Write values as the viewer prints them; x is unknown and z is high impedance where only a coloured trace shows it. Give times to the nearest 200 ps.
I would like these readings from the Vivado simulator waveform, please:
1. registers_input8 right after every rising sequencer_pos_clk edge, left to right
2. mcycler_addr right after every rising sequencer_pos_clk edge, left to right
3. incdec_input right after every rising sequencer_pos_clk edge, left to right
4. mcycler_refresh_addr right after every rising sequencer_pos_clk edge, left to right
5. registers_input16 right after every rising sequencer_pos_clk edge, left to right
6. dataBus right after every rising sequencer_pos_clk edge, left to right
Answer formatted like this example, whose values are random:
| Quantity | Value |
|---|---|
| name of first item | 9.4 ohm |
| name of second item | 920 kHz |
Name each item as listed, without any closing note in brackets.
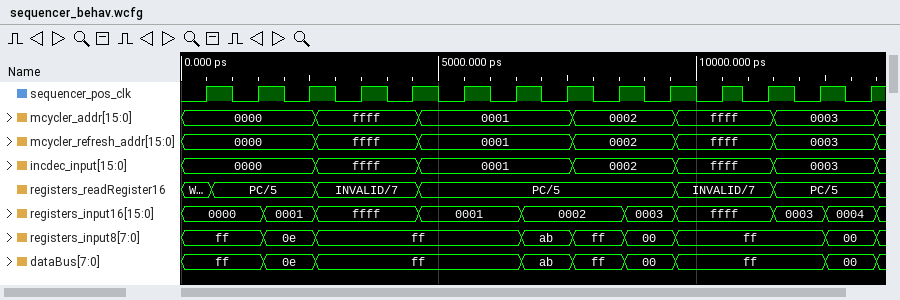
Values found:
| Quantity | Value |
|---|---|
| registers_input8 right after every rising sequencer_pos_clk edge, left to right | ff, ff, 0e, ff, ff, ff, ff, ab, ff, 00, ff, ff, ff, 00 |
| mcycler_addr right after every rising sequencer_pos_clk edge, left to right | 0000, 0000, 0000, ffff, ffff, 0001, 0001, 0001, 0002, 0002, ffff, ffff, 0003, 0003 |
| incdec_input right after every rising sequencer_pos_clk edge, left to right | 0000, 0000, 0000, ffff, ffff, 0001, 0001, 0001, 0002, 0002, ffff, ffff, 0003, 0003 |
| mcycler_refresh_addr right after every rising sequencer_pos_clk edge, left to right | 0000, 0000, 0000, ffff, ffff, 0001, 0001, 0001, 0002, 0002, ffff, ffff, 0003, 0003 |
| registers_input16 right after every rising sequencer_pos_clk edge, left to right | 0000, 0000, 0001, ffff, ffff, 0001, 0001, 0002, 0002, 0003, ffff, ffff, 0003, 0004 |
| dataBus right after every rising sequencer_pos_clk edge, left to right | ff, ff, 0e, ff, ff, ff, ff, ab, ff, 00, ff, ff, ff, 00 |
